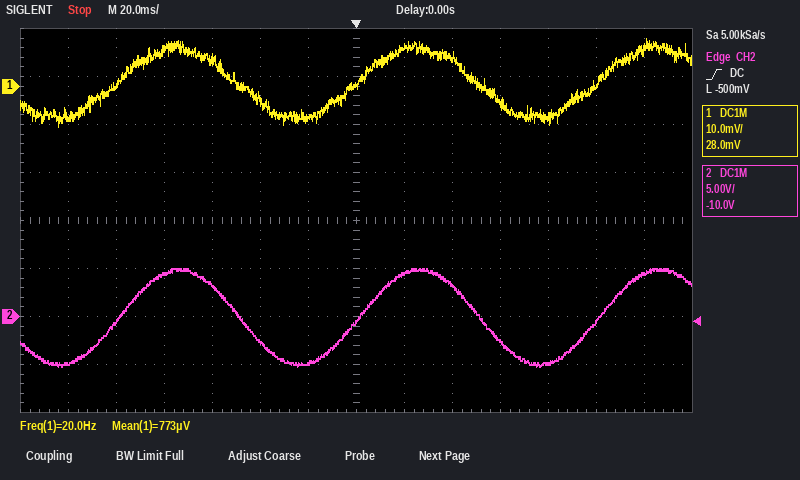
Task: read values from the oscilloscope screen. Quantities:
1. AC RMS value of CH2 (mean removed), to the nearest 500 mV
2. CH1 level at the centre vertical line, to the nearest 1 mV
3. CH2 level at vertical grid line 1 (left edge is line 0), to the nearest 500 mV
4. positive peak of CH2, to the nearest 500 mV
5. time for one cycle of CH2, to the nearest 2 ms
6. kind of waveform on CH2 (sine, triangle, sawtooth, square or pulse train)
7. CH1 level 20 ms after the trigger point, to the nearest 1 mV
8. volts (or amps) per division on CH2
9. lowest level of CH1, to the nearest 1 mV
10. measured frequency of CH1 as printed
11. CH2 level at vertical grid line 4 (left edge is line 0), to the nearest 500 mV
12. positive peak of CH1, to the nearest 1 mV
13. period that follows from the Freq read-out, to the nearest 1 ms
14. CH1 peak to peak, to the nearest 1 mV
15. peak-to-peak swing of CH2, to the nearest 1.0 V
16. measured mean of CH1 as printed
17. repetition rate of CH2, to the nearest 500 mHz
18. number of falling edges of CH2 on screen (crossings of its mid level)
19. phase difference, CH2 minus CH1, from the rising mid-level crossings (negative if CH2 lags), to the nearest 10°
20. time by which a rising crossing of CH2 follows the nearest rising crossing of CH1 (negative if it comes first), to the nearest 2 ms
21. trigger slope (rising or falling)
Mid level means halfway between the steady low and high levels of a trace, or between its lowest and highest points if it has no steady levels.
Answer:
3.5 V
0 mV
-5.0 V
5.0 V
100 ms
sine
8 mV
5 V
-8 mV
20.0 Hz
3.5 V
10 mV
50 ms
18 mV
10.0 V
773 µV
10.0 Hz
2
0°
0 ms
rising
